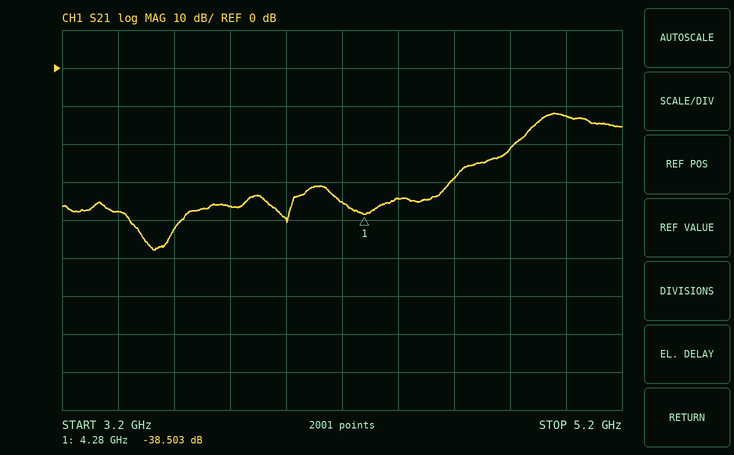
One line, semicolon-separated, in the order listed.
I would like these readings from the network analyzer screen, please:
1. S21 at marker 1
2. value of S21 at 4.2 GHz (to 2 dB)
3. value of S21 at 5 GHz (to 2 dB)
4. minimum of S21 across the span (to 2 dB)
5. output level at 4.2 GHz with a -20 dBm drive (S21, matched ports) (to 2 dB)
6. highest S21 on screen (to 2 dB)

-38.503 dB; -36 dB; -12 dB; -48 dB; -56 dBm; -12 dB
